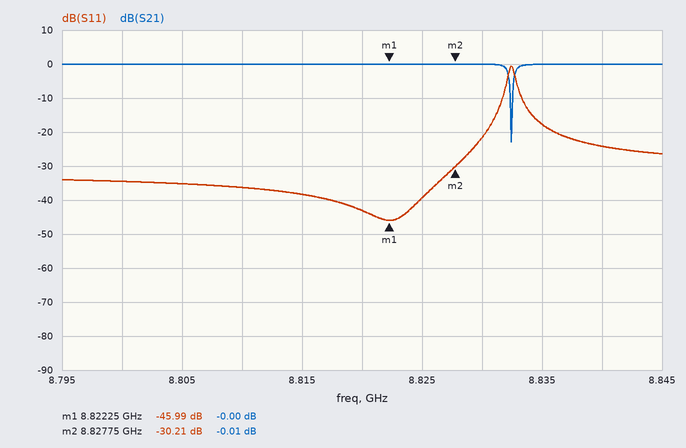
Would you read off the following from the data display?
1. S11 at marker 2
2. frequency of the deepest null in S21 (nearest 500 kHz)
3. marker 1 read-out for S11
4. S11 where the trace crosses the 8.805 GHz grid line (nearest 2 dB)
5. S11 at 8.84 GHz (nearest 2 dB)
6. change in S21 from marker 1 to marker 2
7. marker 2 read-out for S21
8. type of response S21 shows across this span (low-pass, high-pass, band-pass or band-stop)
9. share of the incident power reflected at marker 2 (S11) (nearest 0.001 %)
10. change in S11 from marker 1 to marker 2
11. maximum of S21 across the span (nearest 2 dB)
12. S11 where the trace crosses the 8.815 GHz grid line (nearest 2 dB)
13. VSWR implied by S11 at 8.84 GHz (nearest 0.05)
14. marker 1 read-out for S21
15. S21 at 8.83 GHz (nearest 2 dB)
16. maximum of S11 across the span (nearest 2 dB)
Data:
-30.21 dB
8.8325 GHz
-45.99 dB
-36 dB
-24 dB
-0.01 dB
-0.01 dB
band-stop
0.095 %
15.78 dB
0 dB
-38 dB
1.15
-0.00 dB
0 dB
0 dB
